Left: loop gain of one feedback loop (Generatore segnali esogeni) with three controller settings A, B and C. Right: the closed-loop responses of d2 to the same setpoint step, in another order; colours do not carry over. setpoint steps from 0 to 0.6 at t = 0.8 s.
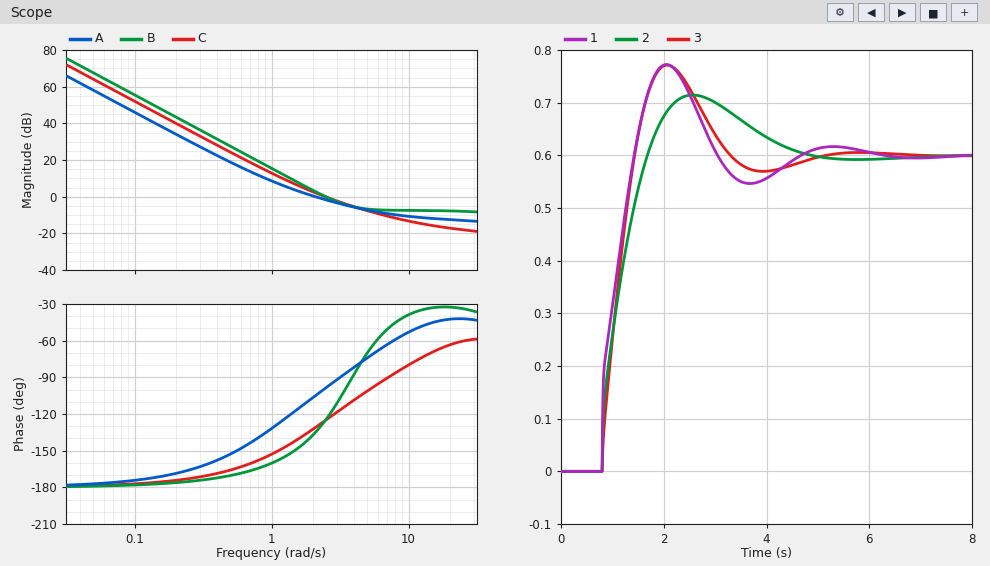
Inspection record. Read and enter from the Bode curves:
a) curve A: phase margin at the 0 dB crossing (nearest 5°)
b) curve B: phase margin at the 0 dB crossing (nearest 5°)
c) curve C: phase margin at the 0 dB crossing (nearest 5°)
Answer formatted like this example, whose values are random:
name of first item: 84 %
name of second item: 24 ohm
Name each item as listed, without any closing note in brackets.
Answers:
curve A: phase margin at the 0 dB crossing: 75°
curve B: phase margin at the 0 dB crossing: 55°
curve C: phase margin at the 0 dB crossing: 55°
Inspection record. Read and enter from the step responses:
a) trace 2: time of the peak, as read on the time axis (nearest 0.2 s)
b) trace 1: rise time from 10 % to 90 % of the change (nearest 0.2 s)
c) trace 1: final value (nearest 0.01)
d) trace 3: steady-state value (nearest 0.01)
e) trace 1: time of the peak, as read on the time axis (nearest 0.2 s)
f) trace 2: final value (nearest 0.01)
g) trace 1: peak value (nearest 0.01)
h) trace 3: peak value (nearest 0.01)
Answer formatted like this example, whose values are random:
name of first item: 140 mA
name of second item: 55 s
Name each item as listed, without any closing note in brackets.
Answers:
trace 2: time of the peak, as read on the time axis: 2.6 s
trace 1: rise time from 10 % to 90 % of the change: 0.6 s
trace 1: final value: 0.60
trace 3: steady-state value: 0.60
trace 1: time of the peak, as read on the time axis: 2.0 s
trace 2: final value: 0.60
trace 1: peak value: 0.77
trace 3: peak value: 0.77
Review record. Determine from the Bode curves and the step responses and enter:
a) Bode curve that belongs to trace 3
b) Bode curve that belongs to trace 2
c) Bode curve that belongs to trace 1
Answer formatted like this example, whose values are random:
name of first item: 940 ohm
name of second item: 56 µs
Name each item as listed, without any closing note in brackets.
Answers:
Bode curve that belongs to trace 3: C
Bode curve that belongs to trace 2: A
Bode curve that belongs to trace 1: B
